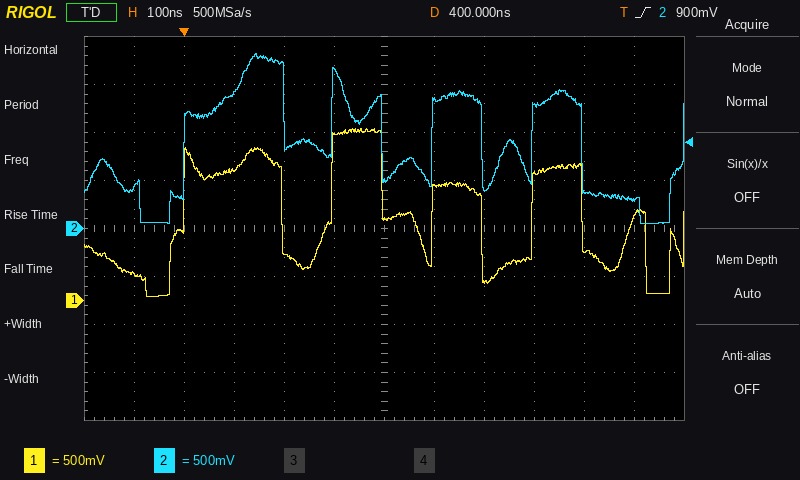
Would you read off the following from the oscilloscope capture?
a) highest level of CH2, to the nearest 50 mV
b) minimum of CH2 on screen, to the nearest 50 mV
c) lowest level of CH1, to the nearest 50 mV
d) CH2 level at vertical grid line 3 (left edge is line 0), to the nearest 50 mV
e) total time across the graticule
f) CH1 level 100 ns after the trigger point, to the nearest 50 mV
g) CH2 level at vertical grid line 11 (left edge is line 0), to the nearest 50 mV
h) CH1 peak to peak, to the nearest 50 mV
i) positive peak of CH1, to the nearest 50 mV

1.80 V
50 mV
50 mV
1.40 V
1.2 µs
1.35 V
300 mV
1.75 V
1.80 V
